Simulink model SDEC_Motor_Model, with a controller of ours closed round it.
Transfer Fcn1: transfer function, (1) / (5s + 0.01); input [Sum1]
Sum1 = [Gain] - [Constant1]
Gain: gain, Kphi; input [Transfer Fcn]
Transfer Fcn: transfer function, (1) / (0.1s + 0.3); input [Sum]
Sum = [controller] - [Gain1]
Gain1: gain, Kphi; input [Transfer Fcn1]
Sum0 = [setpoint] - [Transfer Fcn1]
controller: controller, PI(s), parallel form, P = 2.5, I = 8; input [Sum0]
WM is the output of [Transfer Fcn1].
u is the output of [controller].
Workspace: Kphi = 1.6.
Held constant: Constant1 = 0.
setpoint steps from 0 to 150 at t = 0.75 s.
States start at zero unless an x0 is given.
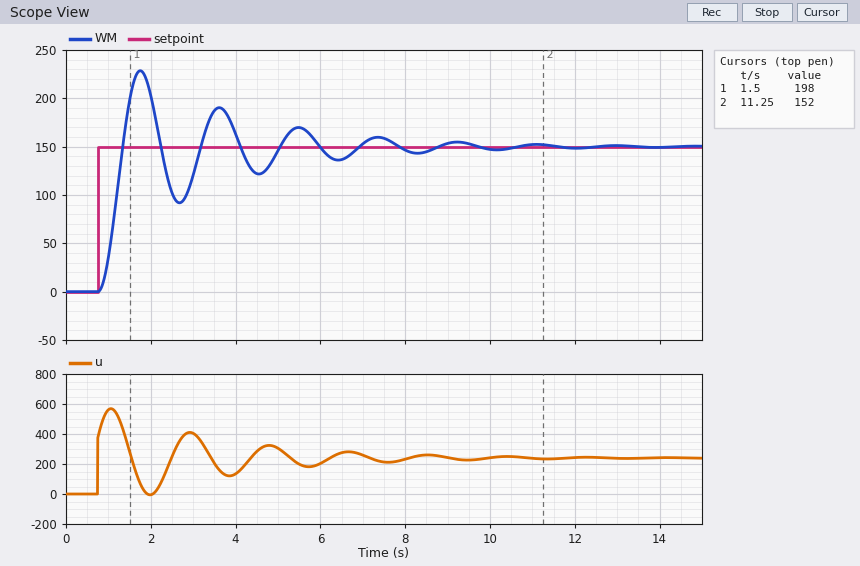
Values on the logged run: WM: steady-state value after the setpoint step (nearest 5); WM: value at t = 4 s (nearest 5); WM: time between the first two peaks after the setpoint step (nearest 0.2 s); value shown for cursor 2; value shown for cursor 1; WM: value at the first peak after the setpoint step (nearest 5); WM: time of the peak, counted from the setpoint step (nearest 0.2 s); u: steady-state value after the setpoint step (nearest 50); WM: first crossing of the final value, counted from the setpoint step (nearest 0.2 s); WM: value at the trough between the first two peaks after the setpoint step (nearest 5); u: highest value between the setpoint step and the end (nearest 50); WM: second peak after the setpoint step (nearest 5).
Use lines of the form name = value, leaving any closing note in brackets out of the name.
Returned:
WM: steady-state value after the setpoint step = 150
WM: value at t = 4 s = 165
WM: time between the first two peaks after the setpoint step = 1.8 s
value shown for cursor 2 = 152
value shown for cursor 1 = 198
WM: value at the first peak after the setpoint step = 230
WM: time of the peak, counted from the setpoint step = 1.0 s
u: steady-state value after the setpoint step = 250
WM: first crossing of the final value, counted from the setpoint step = 0.6 s
WM: value at the trough between the first two peaks after the setpoint step = 90
u: highest value between the setpoint step and the end = 550
WM: second peak after the setpoint step = 190
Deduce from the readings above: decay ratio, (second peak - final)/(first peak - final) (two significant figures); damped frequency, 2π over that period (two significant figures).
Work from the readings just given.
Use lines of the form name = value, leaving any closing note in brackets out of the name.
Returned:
decay ratio, (second peak - final)/(first peak - final) = 0.50
damped frequency, 2π over that period = 3.5 rad/s
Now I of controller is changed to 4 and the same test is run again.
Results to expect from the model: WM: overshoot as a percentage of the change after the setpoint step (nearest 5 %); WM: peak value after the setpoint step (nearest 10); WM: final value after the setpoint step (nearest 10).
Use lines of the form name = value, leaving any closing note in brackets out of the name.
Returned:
WM: overshoot as a percentage of the change after the setpoint step = 20 %
WM: peak value after the setpoint step = 180
WM: final value after the setpoint step = 150
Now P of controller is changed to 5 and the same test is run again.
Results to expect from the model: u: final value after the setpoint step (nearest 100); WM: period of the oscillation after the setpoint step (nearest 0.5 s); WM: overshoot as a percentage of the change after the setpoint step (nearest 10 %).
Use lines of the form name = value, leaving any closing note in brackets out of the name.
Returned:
u: final value after the setpoint step = 200
WM: period of the oscillation after the setpoint step = 1.5 s
WM: overshoot as a percentage of the change after the setpoint step = 40 %
